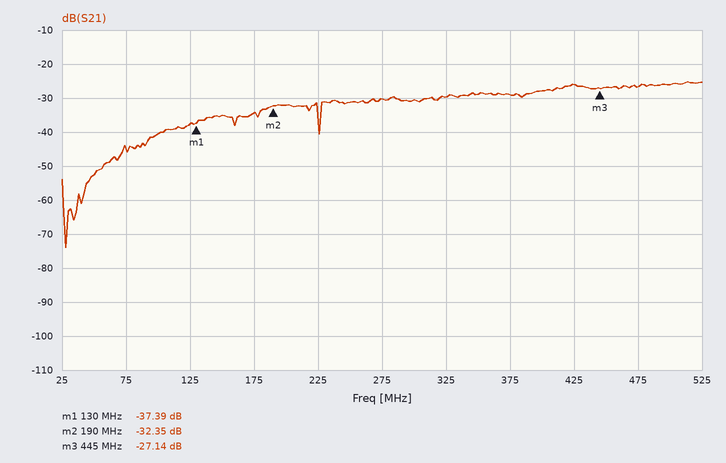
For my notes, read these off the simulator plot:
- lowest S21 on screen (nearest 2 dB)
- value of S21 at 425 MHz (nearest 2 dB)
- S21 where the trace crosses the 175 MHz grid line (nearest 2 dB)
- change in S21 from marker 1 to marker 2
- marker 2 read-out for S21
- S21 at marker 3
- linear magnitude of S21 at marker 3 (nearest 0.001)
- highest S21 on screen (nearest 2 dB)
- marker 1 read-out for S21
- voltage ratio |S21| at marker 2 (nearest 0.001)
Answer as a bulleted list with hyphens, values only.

- -74 dB
- -26 dB
- -34 dB
- 5.04 dB
- -32.35 dB
- -27.14 dB
- 0.044
- -26 dB
- -37.39 dB
- 0.024
